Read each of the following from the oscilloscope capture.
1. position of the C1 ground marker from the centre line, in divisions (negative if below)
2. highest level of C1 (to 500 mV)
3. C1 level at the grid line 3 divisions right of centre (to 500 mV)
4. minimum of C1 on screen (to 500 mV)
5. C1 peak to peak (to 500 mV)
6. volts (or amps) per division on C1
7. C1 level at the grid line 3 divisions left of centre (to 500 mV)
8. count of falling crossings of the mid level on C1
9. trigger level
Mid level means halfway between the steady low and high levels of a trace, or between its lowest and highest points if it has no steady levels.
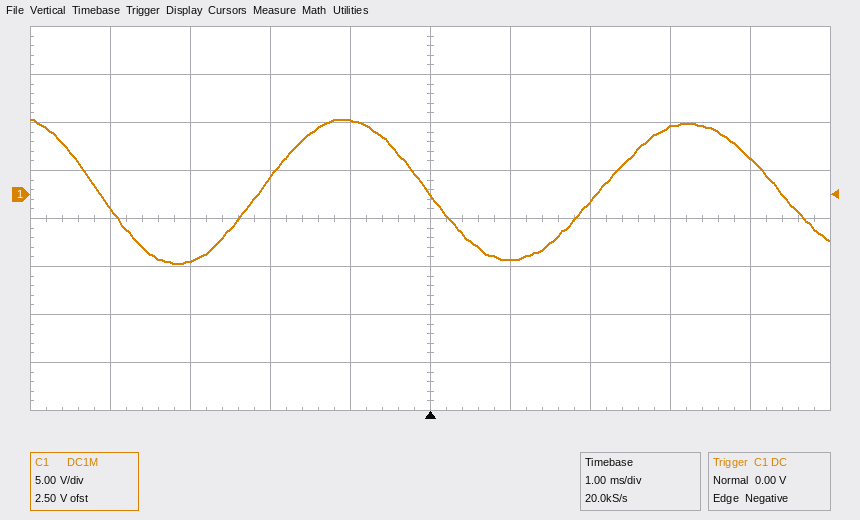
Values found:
+0.5 div
8.0 V
7.0 V
-7.0 V
15.0 V
5 V
-7.0 V
3
0.00 V
